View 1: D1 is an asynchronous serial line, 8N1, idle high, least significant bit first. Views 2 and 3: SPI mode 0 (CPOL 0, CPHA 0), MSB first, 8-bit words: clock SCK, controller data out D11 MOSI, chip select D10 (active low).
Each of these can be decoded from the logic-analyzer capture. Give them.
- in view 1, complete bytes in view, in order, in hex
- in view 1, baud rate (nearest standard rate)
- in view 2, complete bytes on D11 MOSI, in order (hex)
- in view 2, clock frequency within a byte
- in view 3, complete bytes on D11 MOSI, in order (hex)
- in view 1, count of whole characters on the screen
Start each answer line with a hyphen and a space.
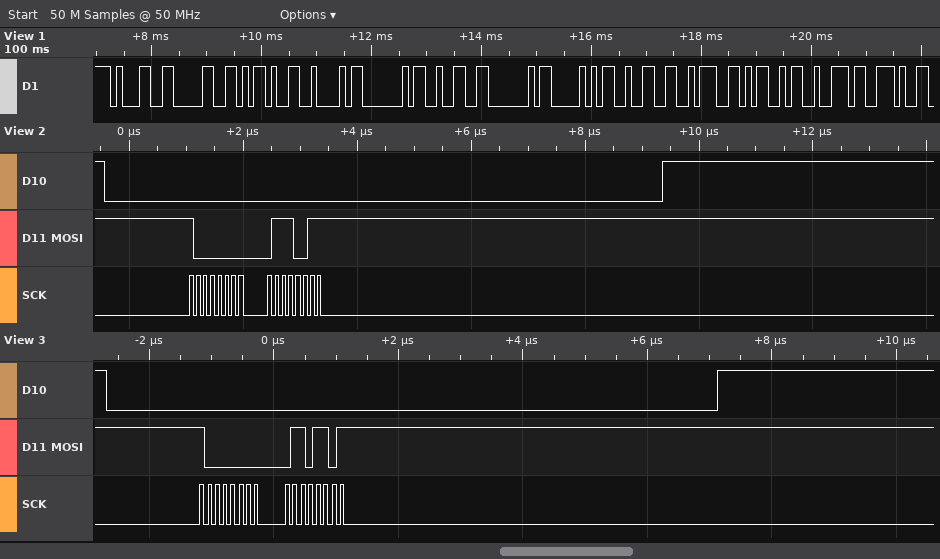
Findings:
- 31 30 2D 42 40 32 40 50 32 3A 4D 72 2E
- 9600 baud
- 0x80 0x73
- 8 MHz
- 80 6D
- 13
